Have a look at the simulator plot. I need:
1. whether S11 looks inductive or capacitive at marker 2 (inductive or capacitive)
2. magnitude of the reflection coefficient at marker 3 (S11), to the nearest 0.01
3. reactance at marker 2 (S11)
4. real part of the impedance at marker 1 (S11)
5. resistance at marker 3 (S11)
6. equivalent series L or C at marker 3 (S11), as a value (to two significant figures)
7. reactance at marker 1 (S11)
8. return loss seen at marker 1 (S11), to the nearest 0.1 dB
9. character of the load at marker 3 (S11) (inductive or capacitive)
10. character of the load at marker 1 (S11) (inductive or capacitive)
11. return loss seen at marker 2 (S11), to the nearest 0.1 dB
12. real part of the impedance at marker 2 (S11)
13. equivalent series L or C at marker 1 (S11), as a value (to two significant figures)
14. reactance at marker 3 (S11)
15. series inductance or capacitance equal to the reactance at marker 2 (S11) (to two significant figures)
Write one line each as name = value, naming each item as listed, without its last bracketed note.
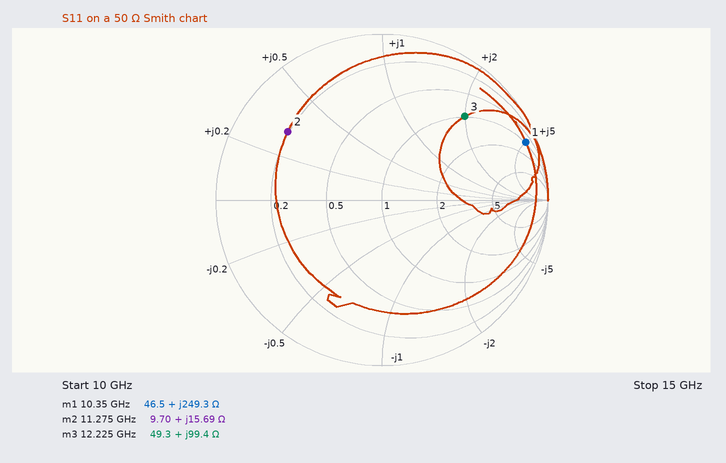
whether S11 looks inductive or capacitive at marker 2 = inductive
magnitude of the reflection coefficient at marker 3 (S11), to the nearest 0.01 = 0.71
reactance at marker 2 = +15.69 Ω
real part of the impedance at marker 1 = 46.5 Ω
resistance at marker 3 = 49.3 Ω
equivalent series L or C at marker 3 (S11), as a value = 1.3 nH
reactance at marker 1 = +249.3 Ω
return loss seen at marker 1 (S11), to the nearest 0.1 dB = 0.6 dB
character of the load at marker 3 (S11) = inductive
character of the load at marker 1 (S11) = inductive
return loss seen at marker 2 (S11), to the nearest 0.1 dB = 3.1 dB
real part of the impedance at marker 2 = 9.70 Ω
equivalent series L or C at marker 1 (S11), as a value = 3.8 nH
reactance at marker 3 = +99.4 Ω
series inductance or capacitance equal to the reactance at marker 2 (S11) = 220 pH
